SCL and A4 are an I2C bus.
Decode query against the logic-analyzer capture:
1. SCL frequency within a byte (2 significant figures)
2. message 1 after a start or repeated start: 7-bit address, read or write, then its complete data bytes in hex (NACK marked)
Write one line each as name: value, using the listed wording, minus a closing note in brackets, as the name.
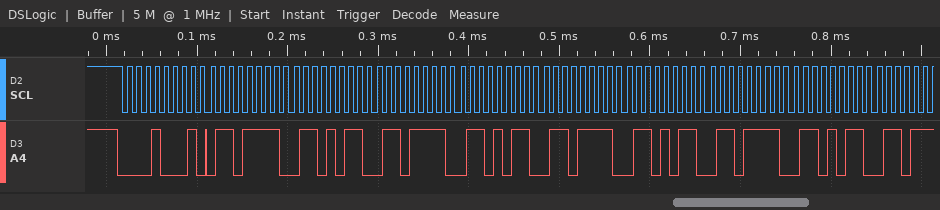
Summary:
SCL frequency within a byte: 100 kHz
message 1 after a start or repeated start: 7-bit address, read or write, then its complete data bytes in hex: 0x08 read: 6F 6B 6F 6B 6F 6B 6F 6B
